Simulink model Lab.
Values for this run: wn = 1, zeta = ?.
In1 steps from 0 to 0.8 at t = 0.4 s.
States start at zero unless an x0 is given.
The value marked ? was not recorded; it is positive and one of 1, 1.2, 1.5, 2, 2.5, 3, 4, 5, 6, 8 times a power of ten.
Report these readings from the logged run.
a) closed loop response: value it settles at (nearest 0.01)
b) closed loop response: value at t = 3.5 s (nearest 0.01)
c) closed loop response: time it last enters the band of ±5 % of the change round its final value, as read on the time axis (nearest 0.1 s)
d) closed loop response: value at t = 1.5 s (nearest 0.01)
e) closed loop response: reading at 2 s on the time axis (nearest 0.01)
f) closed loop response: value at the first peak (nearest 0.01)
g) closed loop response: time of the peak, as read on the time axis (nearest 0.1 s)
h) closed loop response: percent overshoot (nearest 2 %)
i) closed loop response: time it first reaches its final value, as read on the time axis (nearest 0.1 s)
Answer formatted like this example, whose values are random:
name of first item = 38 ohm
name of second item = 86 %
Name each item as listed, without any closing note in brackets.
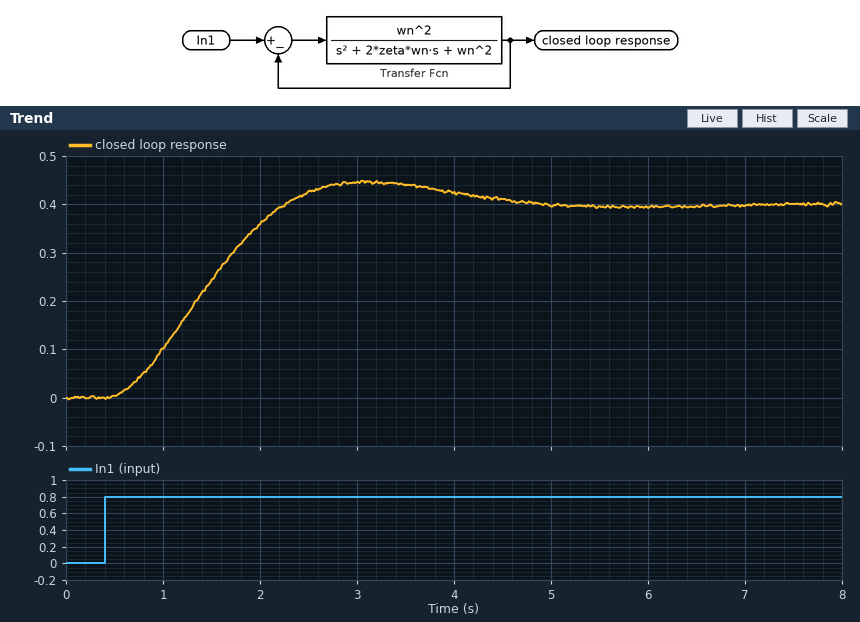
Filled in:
closed loop response: value it settles at = 0.40
closed loop response: value at t = 3.5 s = 0.44
closed loop response: time it last enters the band of ±5 % of the change round its final value, as read on the time axis = 4.1 s
closed loop response: value at t = 1.5 s = 0.24
closed loop response: reading at 2 s on the time axis = 0.36
closed loop response: value at the first peak = 0.45
closed loop response: time of the peak, as read on the time axis = 3.1 s
closed loop response: percent overshoot = 12 %
closed loop response: time it first reaches its final value, as read on the time axis = 2.3 s
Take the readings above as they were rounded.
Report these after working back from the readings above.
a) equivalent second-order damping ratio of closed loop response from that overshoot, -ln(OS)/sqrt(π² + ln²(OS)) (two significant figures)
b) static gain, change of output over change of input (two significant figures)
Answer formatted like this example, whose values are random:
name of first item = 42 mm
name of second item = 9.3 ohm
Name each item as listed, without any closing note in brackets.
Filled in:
equivalent second-order damping ratio of closed loop response from that overshoot, -ln(OS)/sqrt(π² + ln²(OS)) = 0.56
static gain, change of output over change of input = 0.50
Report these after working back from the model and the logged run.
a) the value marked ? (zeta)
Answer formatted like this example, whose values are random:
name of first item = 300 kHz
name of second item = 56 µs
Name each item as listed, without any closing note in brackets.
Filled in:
the value marked ? = 0.8
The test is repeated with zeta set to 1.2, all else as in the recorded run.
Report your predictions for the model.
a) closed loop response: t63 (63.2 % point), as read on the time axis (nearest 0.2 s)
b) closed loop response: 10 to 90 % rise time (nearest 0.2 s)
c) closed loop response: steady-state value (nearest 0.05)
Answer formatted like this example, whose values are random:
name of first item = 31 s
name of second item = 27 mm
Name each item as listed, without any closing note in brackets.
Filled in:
closed loop response: t63 (63.2 % point), as read on the time axis = 1.8 s
closed loop response: 10 to 90 % rise time = 1.8 s
closed loop response: steady-state value = 0.40
